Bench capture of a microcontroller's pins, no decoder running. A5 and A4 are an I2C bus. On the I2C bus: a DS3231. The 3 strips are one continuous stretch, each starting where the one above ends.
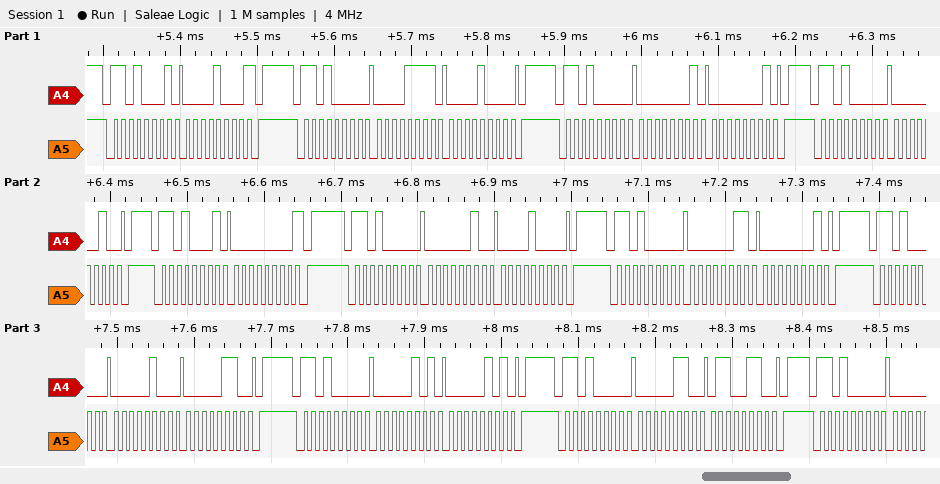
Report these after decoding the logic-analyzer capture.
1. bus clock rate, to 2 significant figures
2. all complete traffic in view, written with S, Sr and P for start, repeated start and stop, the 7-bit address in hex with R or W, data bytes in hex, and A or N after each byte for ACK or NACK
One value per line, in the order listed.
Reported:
100 kHz
S 68R A 08 N P S 68W A 0F A 08 A P S 68W A 01 A 01 A P S 68W A 02 A P S 68R A 00 N P S 68W A 02 A 08 A P S 68W A 03 A 01 A P S 68W A 04 A 06 A P S 68W A 05 A 05 A P S 68W A 06 A 66 A P S 68W A
